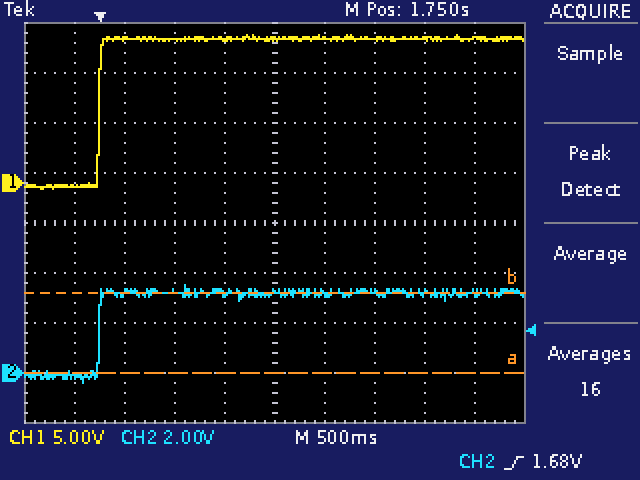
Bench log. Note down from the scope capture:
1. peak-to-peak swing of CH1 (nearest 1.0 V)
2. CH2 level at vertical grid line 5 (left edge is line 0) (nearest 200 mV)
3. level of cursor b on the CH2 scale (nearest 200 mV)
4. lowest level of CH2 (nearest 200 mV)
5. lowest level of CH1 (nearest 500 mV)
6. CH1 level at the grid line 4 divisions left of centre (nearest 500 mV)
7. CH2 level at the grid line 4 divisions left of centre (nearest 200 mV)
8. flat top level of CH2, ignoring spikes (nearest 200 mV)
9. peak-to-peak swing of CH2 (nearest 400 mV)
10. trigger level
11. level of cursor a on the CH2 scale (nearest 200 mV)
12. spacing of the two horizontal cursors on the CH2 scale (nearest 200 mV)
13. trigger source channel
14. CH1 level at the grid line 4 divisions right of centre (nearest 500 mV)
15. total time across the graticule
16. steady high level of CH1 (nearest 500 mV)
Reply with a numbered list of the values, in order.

1. 15.0 V
2. 3.2 V
3. 3.2 V
4. -400 mV
5. -500 mV
6. -500 mV
7. -200 mV
8. 3.2 V
9. 4.0 V
10. 1.68 V
11. 0.0 V
12. 3.2 V
13. CH2
14. 14.5 V
15. 5 s
16. 14.5 V
